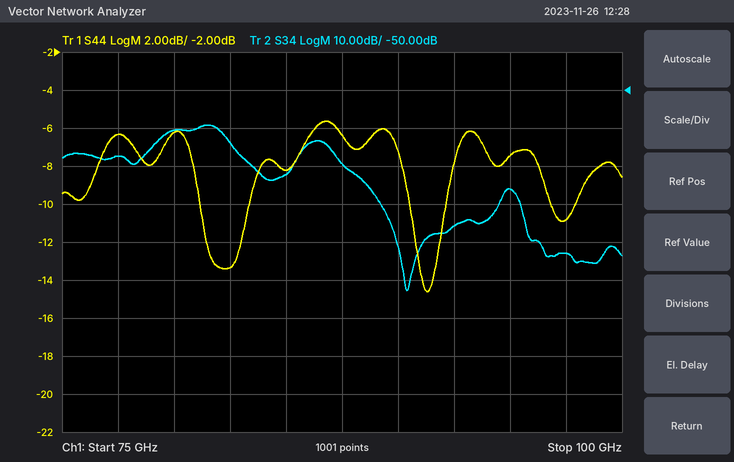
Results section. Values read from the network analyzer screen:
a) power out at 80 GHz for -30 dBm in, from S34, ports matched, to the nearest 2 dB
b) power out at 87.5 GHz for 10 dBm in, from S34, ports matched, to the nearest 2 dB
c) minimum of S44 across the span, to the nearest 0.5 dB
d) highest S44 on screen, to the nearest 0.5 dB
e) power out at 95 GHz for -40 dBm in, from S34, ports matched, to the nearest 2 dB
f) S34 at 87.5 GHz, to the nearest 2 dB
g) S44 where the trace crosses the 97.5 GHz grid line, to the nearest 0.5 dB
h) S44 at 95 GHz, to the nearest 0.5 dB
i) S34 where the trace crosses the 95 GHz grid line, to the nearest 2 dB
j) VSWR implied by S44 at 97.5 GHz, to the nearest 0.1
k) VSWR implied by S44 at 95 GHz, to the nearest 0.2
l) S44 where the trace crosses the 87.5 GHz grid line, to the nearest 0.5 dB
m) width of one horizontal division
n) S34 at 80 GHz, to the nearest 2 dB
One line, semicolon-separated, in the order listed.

-90 dBm; -60 dBm; -14.5 dB; -5.5 dB; -116 dBm; -70 dB; -11.0 dB; -7.5 dB; -76 dB; 1.8; 2.4; -6.5 dB; 2.5 GHz; -60 dB
